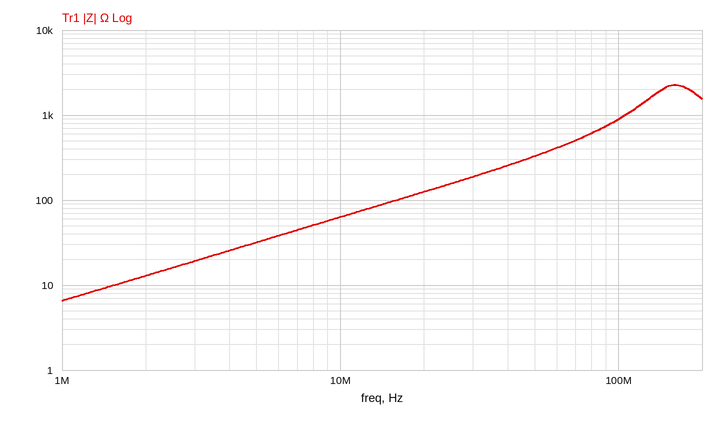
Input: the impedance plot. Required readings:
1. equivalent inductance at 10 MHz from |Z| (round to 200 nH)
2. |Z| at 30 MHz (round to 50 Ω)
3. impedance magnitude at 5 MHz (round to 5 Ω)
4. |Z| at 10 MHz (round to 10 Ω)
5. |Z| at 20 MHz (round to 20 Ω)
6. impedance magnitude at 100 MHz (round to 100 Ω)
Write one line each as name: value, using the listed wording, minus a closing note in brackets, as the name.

equivalent inductance at 10 MHz from |Z|: 1.0 µH
|Z| at 30 MHz: 200 Ω
impedance magnitude at 5 MHz: 30 Ω
|Z| at 10 MHz: 60 Ω
|Z| at 20 MHz: 120 Ω
impedance magnitude at 100 MHz: 900 Ω
